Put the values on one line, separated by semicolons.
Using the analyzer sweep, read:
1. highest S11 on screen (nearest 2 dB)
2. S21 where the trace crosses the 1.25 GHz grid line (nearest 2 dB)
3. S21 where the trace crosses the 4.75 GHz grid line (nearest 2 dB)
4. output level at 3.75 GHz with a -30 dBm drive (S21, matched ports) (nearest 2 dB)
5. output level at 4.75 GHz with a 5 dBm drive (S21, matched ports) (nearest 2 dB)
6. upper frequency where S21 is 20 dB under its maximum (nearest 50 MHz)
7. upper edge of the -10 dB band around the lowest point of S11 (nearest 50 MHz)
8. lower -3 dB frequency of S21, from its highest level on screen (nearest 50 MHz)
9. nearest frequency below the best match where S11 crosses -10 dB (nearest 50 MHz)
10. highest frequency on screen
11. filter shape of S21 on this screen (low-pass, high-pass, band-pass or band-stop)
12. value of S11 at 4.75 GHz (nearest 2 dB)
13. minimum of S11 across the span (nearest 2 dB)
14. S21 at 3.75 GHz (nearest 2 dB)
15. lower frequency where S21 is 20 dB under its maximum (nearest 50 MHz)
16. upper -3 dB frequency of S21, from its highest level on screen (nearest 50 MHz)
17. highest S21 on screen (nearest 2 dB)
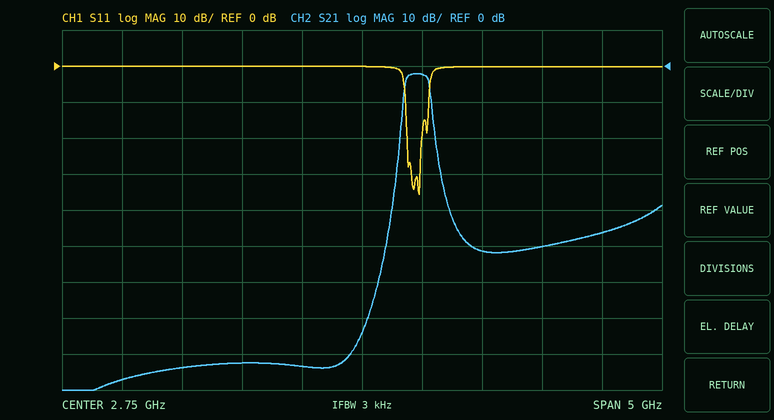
0 dB; -84 dB; -46 dB; -82 dBm; -42 dBm; 3.35 GHz; 3.30 GHz; 3.10 GHz; 3.10 GHz; 5.25 GHz; band-pass; 0 dB; -36 dB; -52 dB; 3.05 GHz; 3.30 GHz; -2 dB
